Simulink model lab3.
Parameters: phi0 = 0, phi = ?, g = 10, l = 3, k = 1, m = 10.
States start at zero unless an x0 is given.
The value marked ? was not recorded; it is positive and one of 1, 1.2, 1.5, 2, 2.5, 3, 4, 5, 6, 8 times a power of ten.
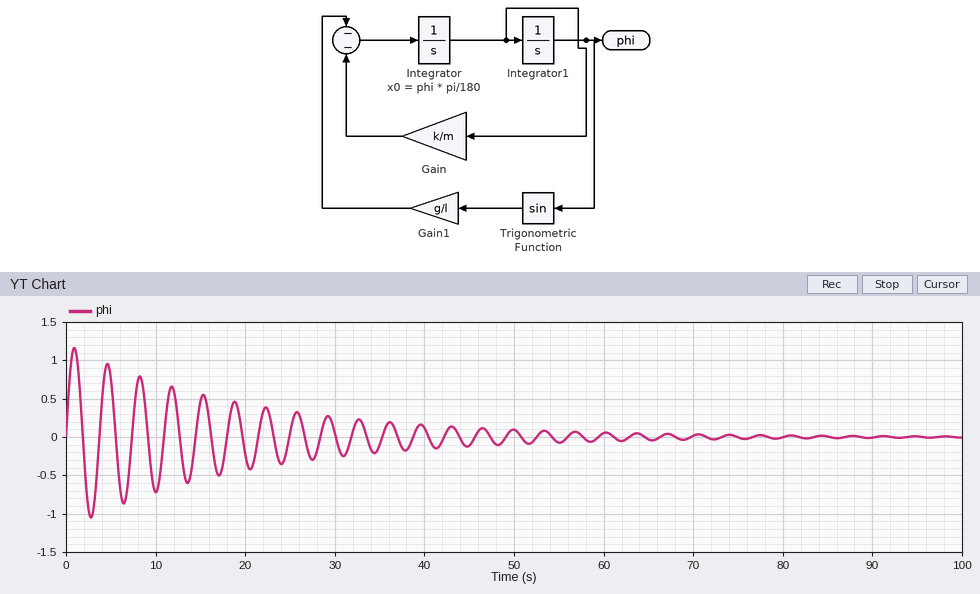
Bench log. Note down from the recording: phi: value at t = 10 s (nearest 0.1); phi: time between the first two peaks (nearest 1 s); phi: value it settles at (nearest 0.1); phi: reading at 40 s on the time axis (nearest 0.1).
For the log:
-0.7
4 s
0.0
0.1
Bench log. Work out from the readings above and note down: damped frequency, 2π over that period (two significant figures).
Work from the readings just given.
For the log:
1.6 rad/s
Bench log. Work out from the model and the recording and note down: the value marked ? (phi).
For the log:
120
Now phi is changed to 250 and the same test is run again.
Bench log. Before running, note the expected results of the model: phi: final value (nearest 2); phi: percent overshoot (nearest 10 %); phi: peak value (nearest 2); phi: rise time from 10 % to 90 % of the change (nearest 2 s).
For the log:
12
20 %
14
6 s
